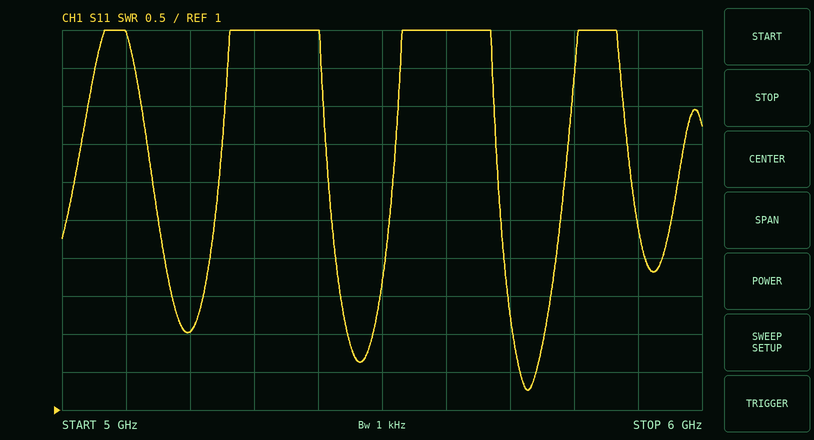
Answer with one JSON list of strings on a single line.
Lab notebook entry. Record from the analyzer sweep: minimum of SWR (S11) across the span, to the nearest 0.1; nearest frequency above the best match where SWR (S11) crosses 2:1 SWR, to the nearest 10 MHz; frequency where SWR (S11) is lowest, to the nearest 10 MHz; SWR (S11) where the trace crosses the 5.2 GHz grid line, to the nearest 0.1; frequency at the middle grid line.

["1.3", "5.75 GHz", "5.73 GHz", "2.0", "5.5 GHz"]
